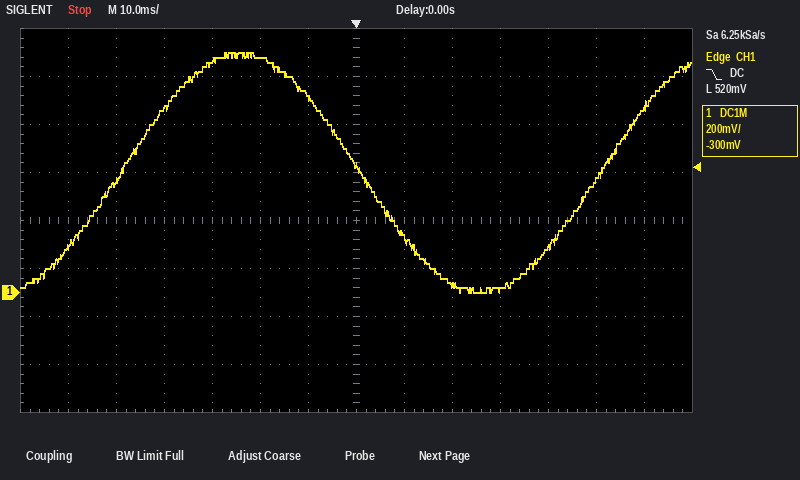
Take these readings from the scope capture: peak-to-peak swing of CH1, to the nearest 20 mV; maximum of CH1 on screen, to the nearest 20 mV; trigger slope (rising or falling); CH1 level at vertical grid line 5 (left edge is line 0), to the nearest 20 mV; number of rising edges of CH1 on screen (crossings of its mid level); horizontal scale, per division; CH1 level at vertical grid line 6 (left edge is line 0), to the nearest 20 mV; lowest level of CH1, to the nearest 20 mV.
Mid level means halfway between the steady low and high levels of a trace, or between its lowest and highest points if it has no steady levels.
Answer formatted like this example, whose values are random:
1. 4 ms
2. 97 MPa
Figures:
1. 1.00 V
2. 1.00 V
3. falling
4. 980 mV
5. 2
6. 10 ms
7. 820 mV
8. 0 mV
